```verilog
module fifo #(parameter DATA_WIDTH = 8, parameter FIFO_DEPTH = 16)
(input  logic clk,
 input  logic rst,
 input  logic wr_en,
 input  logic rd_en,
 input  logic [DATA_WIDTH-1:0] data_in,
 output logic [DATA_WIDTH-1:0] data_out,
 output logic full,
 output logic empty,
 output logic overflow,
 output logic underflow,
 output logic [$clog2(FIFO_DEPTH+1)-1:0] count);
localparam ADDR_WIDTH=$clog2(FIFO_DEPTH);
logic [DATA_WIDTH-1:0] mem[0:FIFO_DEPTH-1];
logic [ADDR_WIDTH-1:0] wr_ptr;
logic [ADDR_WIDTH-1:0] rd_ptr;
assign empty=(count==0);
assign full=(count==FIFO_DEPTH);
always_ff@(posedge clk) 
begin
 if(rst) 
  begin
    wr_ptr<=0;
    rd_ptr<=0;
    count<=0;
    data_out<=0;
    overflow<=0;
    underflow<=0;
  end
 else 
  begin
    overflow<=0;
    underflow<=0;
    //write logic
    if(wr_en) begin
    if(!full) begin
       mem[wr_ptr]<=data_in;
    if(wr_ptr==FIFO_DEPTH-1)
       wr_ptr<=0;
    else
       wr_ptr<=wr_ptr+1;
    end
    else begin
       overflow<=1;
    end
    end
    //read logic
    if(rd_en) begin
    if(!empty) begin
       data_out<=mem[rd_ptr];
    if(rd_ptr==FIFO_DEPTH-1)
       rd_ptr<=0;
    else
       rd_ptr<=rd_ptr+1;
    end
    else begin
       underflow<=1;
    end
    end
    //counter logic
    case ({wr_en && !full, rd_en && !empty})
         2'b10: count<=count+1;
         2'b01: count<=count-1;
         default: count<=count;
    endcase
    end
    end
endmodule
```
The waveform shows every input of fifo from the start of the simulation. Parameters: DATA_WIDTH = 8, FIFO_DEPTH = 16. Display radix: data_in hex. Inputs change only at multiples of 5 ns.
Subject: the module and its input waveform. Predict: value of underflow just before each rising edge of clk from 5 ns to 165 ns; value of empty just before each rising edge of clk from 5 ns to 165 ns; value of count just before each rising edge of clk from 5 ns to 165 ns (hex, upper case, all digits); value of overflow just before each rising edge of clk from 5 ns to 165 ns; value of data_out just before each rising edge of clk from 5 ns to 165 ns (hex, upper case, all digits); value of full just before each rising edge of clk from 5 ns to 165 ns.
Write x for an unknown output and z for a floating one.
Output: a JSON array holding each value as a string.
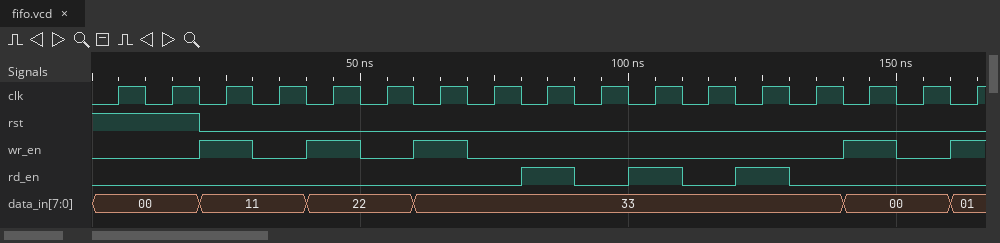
["x 0 0 0 0 0 0 0 0 0 0 0 0 0 0 0 0", "x 1 1 0 0 0 0 0 0 0 0 0 0 1 1 0 0", "x, 00, 00, 01, 01, 02, 02, 03, 03, 02, 02, 01, 01, 00, 00, 01, 01", "x 0 0 0 0 0 0 0 0 0 0 0 0 0 0 0 0", "x, 00, 00, 00, 00, 00, 00, 00, 00, 11, 11, 22, 22, 33, 33, 33, 33", "x 0 0 0 0 0 0 0 0 0 0 0 0 0 0 0 0"]
